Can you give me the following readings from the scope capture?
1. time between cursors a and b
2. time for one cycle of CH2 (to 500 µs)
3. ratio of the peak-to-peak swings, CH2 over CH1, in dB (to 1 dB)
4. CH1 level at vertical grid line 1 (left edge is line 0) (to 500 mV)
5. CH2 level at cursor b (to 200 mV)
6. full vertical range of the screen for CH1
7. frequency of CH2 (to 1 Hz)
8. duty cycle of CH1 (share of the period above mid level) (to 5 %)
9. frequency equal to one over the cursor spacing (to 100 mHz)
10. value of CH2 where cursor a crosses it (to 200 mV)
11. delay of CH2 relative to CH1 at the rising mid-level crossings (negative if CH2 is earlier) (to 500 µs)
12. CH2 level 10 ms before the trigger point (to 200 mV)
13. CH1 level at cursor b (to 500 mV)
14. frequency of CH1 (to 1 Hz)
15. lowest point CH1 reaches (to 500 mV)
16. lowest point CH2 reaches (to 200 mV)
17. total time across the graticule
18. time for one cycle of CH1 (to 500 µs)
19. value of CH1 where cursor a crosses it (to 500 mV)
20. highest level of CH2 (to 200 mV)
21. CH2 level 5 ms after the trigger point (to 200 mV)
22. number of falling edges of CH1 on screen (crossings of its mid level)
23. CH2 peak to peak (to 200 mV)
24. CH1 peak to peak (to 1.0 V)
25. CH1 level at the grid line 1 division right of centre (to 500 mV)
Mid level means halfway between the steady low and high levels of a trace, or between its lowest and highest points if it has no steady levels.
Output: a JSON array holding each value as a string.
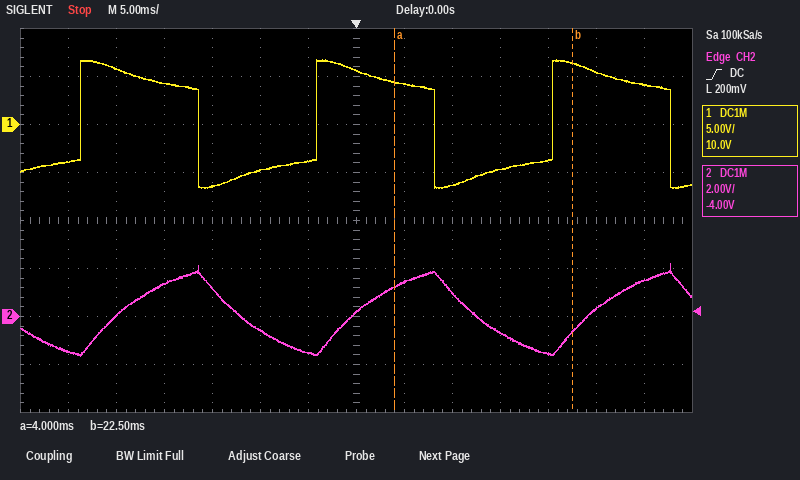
["18.5 ms", "24.5 ms", "-11 dB", "-4.0 V", "-600 mV", "40 V", "41 Hz", "50 %", "54.1 Hz", "1.2 V", "+4.5 ms", "-600 mV", "6.5 V", "41 Hz", "-6.5 V", "-1.6 V", "70 ms", "24.5 ms", "4.5 V", "2.2 V", "1.4 V", "3", "3.8 V", "13.0 V", "4.0 V"]
